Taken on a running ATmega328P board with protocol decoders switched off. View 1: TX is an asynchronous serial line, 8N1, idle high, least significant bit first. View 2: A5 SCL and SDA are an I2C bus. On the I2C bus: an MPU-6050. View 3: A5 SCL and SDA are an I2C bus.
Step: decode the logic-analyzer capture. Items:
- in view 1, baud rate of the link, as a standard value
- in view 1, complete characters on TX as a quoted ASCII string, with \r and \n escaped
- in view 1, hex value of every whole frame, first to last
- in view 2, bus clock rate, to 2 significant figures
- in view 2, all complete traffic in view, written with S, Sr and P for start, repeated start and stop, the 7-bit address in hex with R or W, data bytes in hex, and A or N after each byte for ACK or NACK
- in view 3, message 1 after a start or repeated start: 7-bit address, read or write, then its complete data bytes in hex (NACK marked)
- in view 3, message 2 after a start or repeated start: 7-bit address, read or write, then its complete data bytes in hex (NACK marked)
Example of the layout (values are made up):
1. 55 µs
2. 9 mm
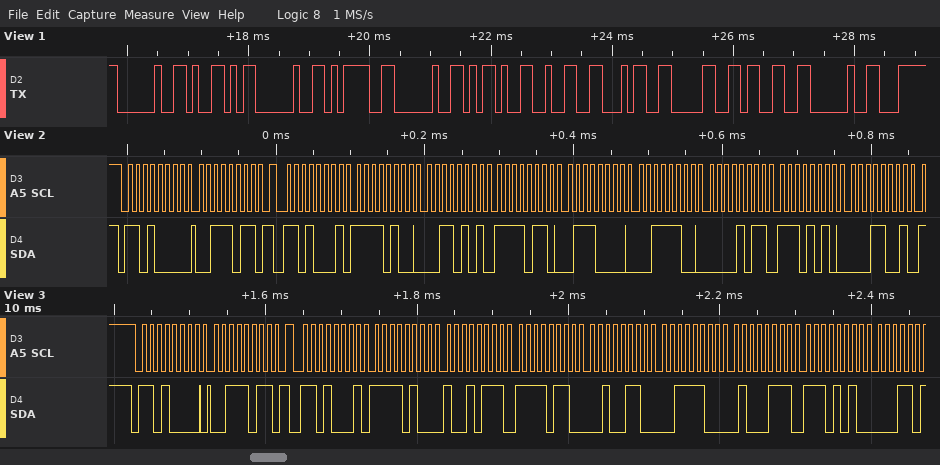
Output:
1. 9600 baud
2. " Y = -2403 "
3. 20 59 20 3D 20 2D 32 34 30 33 20
4. 100 kHz
5. S 68W A 3B A Sr 68R A F4 A 35 A F6 A 70 A 3C A 0B A EA A 19 A
6. 0x68 write: 3B
7. 0x68 read: F4 97 F6 26 3C 47 EA
